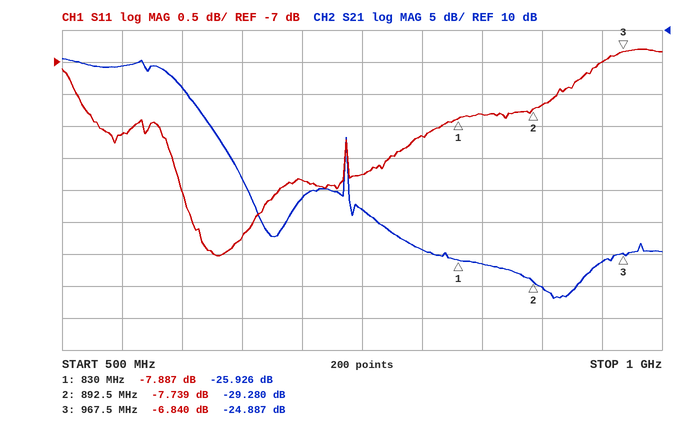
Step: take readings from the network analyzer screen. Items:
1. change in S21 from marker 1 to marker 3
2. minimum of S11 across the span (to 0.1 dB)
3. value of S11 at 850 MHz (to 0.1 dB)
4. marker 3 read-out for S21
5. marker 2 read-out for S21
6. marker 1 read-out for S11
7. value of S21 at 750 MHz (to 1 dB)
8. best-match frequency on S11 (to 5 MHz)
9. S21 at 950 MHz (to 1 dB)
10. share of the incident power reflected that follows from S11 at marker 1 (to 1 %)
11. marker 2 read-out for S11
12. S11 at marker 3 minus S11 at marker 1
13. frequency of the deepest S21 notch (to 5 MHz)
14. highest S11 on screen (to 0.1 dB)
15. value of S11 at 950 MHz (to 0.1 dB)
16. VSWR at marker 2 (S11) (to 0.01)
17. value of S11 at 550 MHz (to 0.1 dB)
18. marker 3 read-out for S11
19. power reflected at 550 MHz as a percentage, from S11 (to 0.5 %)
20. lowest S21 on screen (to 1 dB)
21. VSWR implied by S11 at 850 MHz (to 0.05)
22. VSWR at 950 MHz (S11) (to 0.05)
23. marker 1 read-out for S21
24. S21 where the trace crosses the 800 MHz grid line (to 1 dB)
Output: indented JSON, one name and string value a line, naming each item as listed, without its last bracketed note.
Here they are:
{
  "change in S21 from marker 1 to marker 3": "1.039 dB",
  "minimum of S11 across the span": "-10.0 dB",
  "value of S11 at 850 MHz": "-7.8 dB",
  "marker 3 read-out for S21": "-24.887 dB",
  "marker 2 read-out for S21": "-29.280 dB",
  "marker 1 read-out for S11": "-7.887 dB",
  "value of S21 at 750 MHz": "-18 dB",
  "best-match frequency on S11": "630 MHz",
  "S21 at 950 MHz": "-26 dB",
  "share of the incident power reflected that follows from S11 at marker 1": "16 %",
  "marker 2 read-out for S11": "-7.739 dB",
  "S11 at marker 3 minus S11 at marker 1": "1.047 dB",
  "frequency of the deepest S21 notch": "910 MHz",
  "highest S11 on screen": "-6.8 dB",
  "value of S11 at 950 MHz": "-7.0 dB",
  "VSWR at marker 2 (S11)": "2.39",
  "value of S11 at 550 MHz": "-8.1 dB",
  "marker 3 read-out for S11": "-6.840 dB",
  "power reflected at 550 MHz as a percentage, from S11": "15.5 %",
  "lowest S21 on screen": "-32 dB",
  "VSWR implied by S11 at 850 MHz": "2.35",
  "VSWR at 950 MHz (S11)": "2.60",
  "marker 1 read-out for S21": "-25.926 dB",
  "S21 where the trace crosses the 800 MHz grid line": "-24 dB"
}
